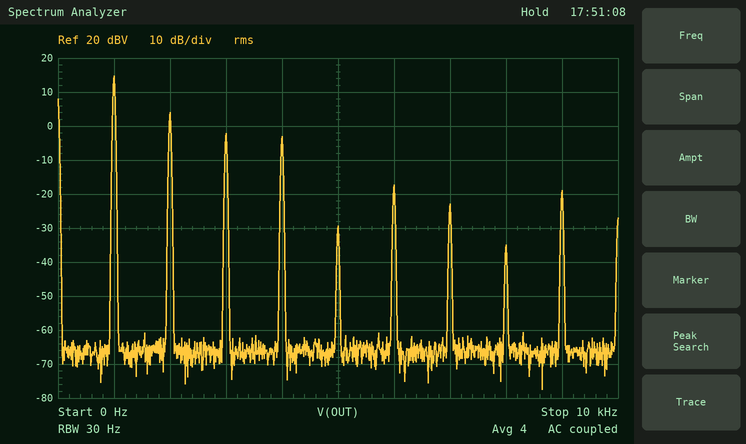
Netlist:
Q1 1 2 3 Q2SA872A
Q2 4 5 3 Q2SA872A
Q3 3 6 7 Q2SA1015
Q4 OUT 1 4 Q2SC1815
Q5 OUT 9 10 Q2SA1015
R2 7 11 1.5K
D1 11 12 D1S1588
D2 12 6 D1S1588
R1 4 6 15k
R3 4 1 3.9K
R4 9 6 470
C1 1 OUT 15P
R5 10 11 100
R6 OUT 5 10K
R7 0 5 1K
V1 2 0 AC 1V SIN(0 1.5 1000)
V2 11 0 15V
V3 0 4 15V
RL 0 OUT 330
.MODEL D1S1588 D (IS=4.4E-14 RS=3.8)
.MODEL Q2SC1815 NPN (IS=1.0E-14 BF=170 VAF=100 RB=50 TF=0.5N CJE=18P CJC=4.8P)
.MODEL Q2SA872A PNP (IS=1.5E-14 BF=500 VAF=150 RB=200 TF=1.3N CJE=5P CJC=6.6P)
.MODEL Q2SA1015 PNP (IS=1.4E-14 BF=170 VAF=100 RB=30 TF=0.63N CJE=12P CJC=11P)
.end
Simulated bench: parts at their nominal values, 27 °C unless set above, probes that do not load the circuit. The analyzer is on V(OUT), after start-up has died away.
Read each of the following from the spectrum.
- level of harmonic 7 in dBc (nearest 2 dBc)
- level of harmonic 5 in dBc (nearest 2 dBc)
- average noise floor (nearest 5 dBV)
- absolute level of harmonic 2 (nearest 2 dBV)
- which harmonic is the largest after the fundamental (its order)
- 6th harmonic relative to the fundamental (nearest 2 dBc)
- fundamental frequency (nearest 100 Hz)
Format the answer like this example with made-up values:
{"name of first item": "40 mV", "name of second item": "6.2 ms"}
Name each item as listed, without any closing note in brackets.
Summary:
{"level of harmonic 7 in dBc": "-38 dBc", "level of harmonic 5 in dBc": "-44 dBc", "average noise floor": "-65 dBV", "absolute level of harmonic 2": "4 dBV", "which harmonic is the largest after the fundamental": "2", "6th harmonic relative to the fundamental": "-32 dBc", "fundamental frequency": "1.0 kHz"}
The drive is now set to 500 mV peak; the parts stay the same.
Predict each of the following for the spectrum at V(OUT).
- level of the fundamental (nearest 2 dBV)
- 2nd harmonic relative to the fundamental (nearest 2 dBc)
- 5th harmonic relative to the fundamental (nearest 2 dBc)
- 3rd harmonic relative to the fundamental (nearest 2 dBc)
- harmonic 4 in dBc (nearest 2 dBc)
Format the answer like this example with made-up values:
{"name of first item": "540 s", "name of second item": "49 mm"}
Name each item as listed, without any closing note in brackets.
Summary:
{"level of the fundamental": "8 dBV", "2nd harmonic relative to the fundamental": "-12 dBc", "5th harmonic relative to the fundamental": "-30 dBc", "3rd harmonic relative to the fundamental": "-22 dBc", "harmonic 4 in dBc": "-38 dBc"}
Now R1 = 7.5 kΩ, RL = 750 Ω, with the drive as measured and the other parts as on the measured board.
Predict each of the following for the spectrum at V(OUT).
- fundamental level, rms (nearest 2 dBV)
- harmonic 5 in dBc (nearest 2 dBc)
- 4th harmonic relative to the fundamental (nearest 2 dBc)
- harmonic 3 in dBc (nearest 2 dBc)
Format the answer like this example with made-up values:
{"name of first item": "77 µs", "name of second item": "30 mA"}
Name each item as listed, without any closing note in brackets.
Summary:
{"fundamental level, rms": "18 dBV", "harmonic 5 in dBc": "-32 dBc", "4th harmonic relative to the fundamental": "-26 dBc", "harmonic 3 in dBc": "-20 dBc"}
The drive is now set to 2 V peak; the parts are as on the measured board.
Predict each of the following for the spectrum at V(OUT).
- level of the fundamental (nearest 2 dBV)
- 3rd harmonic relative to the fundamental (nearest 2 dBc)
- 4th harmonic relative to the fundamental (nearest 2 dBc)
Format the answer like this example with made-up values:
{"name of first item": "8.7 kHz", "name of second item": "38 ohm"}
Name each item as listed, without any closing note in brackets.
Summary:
{"level of the fundamental": "16 dBV", "3rd harmonic relative to the fundamental": "-14 dBc", "4th harmonic relative to the fundamental": "-16 dBc"}
